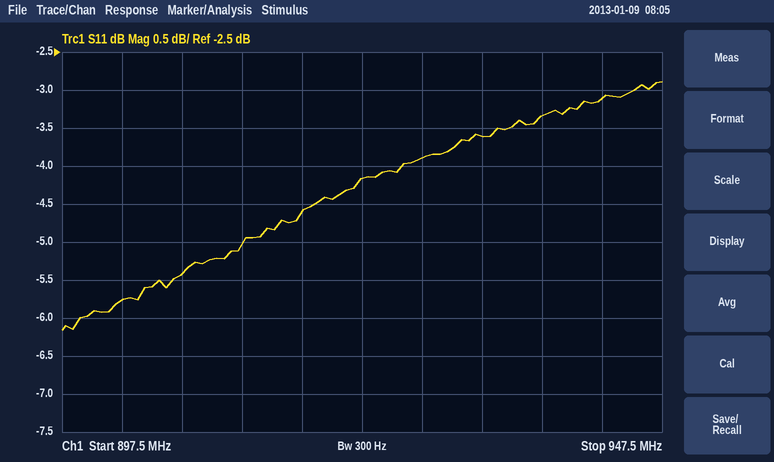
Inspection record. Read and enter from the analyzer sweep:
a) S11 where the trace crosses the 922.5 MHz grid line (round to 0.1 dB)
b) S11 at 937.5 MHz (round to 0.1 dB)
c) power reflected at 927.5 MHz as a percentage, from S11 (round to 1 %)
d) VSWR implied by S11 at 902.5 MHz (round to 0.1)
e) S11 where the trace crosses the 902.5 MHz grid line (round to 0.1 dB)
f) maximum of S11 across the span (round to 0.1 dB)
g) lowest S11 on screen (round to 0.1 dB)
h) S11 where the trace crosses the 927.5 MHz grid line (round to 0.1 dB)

-4.2 dB
-3.3 dB
41 %
3.1
-5.8 dB
-2.9 dB
-6.2 dB
-3.9 dB
